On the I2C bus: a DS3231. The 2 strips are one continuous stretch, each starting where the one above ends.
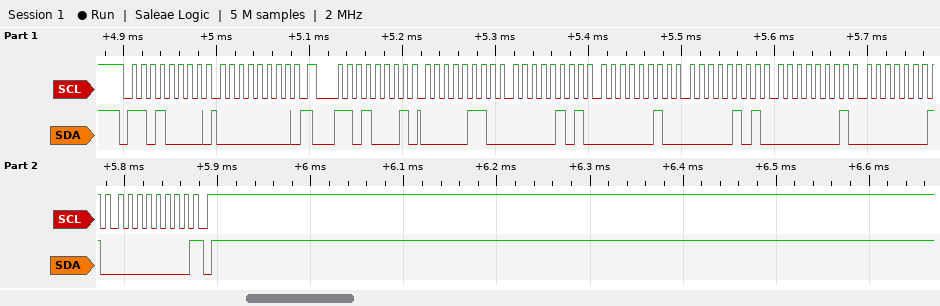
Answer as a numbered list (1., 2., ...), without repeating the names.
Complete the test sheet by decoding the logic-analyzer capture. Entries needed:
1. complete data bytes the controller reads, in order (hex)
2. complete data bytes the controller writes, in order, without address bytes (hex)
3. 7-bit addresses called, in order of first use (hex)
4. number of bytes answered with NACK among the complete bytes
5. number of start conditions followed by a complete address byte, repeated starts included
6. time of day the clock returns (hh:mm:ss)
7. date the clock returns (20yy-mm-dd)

1. 06 05 02 05 01 01 00
2. 00
3. 0x68
4. 1
5. 2
6. 02:05:06
7. 2000-01-01
